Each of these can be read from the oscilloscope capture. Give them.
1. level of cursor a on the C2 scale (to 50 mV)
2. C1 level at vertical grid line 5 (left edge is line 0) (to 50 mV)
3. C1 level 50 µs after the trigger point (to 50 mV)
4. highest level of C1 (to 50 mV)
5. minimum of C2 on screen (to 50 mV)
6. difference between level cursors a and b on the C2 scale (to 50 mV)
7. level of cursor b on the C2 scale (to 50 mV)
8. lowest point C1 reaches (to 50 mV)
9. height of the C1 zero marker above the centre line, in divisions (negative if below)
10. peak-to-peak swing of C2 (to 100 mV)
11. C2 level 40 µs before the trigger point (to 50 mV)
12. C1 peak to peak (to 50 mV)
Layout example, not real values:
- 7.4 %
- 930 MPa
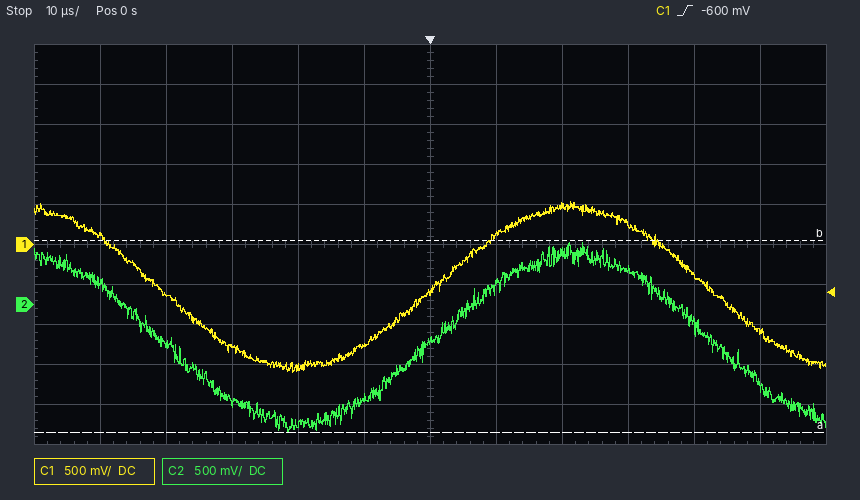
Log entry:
- -1.60 V
- -1.25 V
- -1.10 V
- 550 mV
- -1.60 V
- 2.40 V
- 800 mV
- -1.60 V
- 0.0 div
- 2.40 V
- -500 mV
- 2.15 V
